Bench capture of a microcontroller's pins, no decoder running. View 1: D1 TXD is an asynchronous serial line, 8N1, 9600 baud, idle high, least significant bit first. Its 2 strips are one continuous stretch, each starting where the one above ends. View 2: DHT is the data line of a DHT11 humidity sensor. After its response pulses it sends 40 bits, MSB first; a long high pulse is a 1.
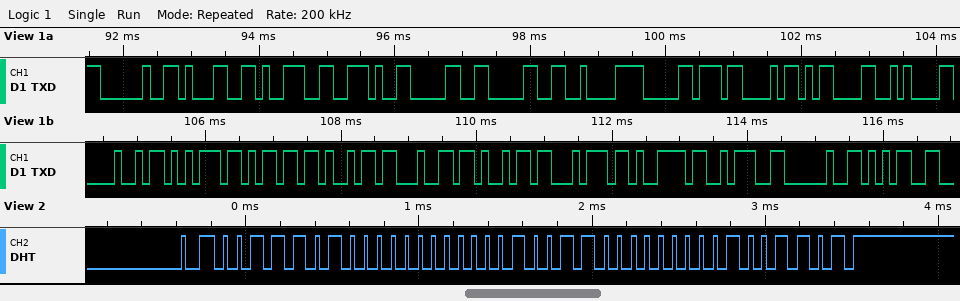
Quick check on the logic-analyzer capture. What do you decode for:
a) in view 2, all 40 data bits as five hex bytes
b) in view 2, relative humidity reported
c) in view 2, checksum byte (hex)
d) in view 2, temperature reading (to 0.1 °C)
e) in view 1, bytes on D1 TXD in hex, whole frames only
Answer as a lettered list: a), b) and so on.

a) 3A 00 13 00 4D
b) 58 %
c) 0x4D
d) 19.0 °C
e) 0x20 0x31 0x39 0x2E 0x30 0x30 0xC2 0xB0 0x43 0x0D 0x0A 0x48 0x75 0x6D 0x69 0x64 0x69 0x74 0x79 0x3A 0x20 0x35
